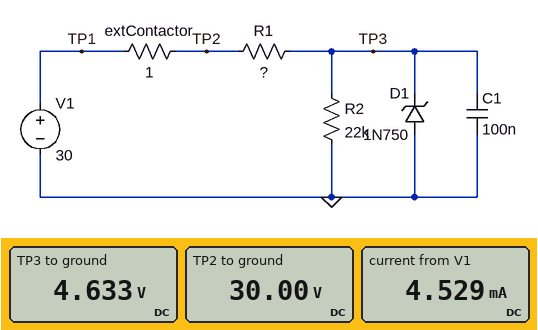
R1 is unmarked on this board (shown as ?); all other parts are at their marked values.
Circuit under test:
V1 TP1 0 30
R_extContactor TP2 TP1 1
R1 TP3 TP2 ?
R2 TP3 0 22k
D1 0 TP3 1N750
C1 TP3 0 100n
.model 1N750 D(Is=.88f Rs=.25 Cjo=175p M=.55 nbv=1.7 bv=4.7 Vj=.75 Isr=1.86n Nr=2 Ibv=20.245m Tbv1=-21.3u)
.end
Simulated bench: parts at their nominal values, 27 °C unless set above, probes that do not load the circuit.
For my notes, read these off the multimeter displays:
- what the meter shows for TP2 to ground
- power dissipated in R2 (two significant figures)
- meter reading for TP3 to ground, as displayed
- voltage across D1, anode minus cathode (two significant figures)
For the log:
30.00 V
980 µW
4.633 V
-4.6 V
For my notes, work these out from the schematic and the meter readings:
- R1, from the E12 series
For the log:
5.6 kΩ
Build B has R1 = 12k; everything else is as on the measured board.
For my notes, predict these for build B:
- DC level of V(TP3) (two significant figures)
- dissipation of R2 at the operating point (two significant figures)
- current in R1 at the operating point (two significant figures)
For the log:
4.6 V
960 µW
2.1 mA
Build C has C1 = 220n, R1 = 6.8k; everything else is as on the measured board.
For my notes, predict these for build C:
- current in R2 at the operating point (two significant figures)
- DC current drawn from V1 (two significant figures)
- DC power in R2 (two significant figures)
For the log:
210 µA
3.7 mA
970 µW
